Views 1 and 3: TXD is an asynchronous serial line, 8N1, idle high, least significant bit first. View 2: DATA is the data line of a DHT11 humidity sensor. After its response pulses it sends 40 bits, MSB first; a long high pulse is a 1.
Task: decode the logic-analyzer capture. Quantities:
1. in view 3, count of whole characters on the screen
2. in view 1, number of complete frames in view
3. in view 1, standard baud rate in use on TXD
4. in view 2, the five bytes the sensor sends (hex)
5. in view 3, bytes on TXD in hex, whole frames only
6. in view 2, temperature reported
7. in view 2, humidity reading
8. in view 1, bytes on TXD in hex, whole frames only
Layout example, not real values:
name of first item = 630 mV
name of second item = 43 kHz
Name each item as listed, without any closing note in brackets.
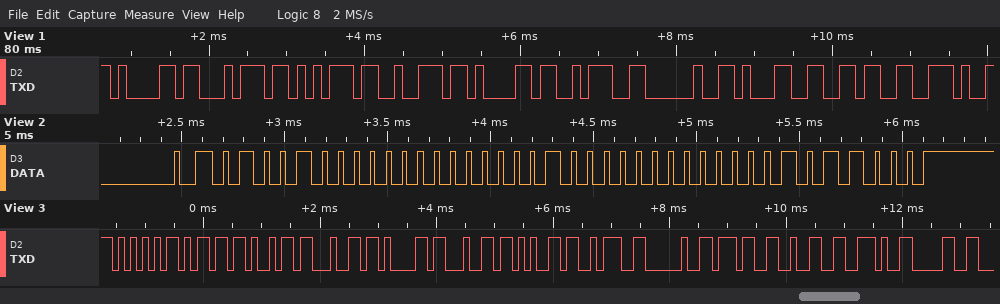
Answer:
in view 3, count of whole characters on the screen = 13
in view 1, number of complete frames in view = 10
in view 1, standard baud rate in use on TXD = 9600 baud
in view 2, the five bytes the sensor sends = 48 00 10 00 58
in view 3, bytes on TXD in hex, whole frames only = 0x55 0x6D 0x69 0x64 0x61 0x64 0x65 0x3A 0x20 0x37 0x32 0x2E 0x30
in view 2, temperature reported = 16.0 °C
in view 2, humidity reading = 72 %
in view 1, bytes on TXD in hex, whole frames only = 61 74 75 72 61 3A 20 31 36 2E
